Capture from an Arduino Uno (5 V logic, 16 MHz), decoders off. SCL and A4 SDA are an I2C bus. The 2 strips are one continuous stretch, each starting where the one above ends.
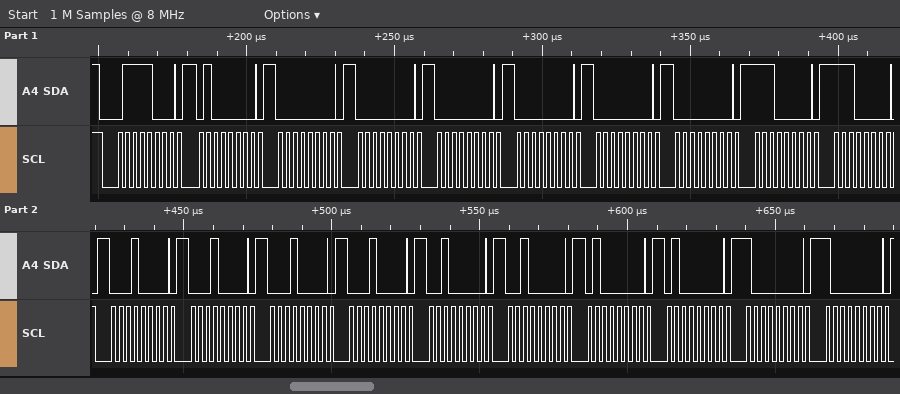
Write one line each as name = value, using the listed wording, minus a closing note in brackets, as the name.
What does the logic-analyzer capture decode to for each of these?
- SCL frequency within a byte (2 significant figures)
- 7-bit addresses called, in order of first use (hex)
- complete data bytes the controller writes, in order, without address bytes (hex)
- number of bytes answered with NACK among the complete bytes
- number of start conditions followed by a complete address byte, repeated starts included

SCL frequency within a byte = 400 kHz
7-bit addresses called, in order of first use = 0x3C
complete data bytes the controller writes, in order, without address bytes = 40 00 00 00 00 00 00 E0 E0 10 10 10 10 20 20 40 40 80 80
number of bytes answered with NACK among the complete bytes = 0
number of start conditions followed by a complete address byte, repeated starts included = 1
